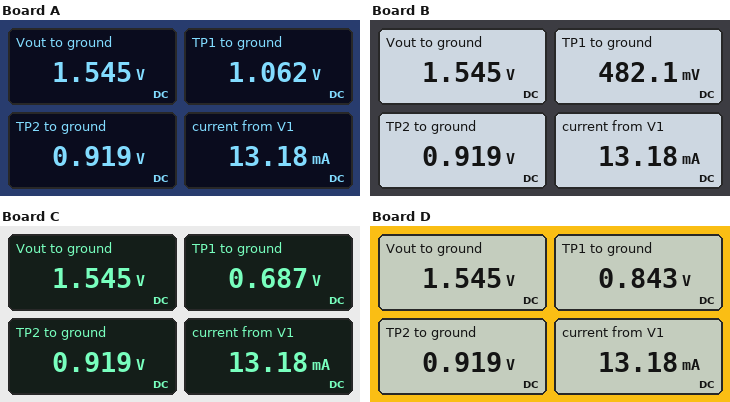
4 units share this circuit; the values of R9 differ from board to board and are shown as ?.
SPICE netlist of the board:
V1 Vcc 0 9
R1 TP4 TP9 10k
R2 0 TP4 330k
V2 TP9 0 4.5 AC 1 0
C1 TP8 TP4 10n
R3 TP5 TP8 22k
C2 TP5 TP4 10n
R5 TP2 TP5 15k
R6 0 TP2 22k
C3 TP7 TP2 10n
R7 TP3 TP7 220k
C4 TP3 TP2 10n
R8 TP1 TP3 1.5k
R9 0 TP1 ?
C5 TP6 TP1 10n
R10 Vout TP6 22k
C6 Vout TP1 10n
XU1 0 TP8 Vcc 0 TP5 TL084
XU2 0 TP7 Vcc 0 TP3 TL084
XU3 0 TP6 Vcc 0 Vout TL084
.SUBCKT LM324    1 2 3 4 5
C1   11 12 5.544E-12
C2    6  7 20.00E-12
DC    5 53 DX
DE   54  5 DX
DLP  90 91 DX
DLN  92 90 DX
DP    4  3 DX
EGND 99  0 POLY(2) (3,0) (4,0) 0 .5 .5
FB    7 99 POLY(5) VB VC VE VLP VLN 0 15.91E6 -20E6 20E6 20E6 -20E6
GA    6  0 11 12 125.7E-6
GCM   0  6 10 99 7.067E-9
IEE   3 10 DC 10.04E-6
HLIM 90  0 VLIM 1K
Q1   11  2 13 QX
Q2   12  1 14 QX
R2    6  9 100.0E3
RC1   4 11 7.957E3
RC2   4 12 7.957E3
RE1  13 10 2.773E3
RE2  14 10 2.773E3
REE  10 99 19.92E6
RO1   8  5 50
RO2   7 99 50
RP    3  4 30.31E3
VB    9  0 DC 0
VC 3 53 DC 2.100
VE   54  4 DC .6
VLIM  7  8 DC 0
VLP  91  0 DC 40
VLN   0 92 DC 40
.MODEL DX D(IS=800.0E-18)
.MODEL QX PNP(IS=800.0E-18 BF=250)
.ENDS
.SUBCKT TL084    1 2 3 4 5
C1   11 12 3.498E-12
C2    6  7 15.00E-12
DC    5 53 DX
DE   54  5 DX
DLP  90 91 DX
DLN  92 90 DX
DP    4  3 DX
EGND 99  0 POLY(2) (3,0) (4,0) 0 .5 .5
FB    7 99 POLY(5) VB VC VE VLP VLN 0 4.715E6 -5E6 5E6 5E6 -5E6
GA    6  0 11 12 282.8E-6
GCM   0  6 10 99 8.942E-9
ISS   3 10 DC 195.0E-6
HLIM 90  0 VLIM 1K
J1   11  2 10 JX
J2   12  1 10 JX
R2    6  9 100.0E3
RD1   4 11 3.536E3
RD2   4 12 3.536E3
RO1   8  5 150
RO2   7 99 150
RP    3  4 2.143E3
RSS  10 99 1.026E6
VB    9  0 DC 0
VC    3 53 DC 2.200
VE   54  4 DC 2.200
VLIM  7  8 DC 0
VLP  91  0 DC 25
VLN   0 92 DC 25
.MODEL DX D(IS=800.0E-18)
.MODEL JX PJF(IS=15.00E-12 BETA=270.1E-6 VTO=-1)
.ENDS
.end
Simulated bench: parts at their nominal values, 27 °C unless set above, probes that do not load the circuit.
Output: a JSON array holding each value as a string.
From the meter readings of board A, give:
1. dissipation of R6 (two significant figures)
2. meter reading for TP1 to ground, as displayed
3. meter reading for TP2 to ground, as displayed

["38 µW", "1.062 V", "0.919 V"]
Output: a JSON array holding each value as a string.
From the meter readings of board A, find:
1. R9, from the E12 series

["3.3 kΩ"]
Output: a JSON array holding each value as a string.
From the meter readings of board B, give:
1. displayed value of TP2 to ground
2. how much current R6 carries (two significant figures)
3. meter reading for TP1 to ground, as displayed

["0.919 V", "42 µA", "482.1 mV"]
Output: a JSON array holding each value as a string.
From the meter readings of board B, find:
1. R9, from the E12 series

["680 Ω"]
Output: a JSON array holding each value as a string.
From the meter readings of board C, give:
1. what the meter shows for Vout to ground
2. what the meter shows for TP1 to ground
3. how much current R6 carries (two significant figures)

["1.545 V", "0.687 V", "42 µA"]
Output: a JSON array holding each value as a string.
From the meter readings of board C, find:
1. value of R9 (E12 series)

["1.2 kΩ"]
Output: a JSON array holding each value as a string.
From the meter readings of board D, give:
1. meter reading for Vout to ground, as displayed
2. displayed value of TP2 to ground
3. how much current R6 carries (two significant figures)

["1.545 V", "0.919 V", "42 µA"]
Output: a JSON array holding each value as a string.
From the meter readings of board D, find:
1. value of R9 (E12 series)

["1.8 kΩ"]
